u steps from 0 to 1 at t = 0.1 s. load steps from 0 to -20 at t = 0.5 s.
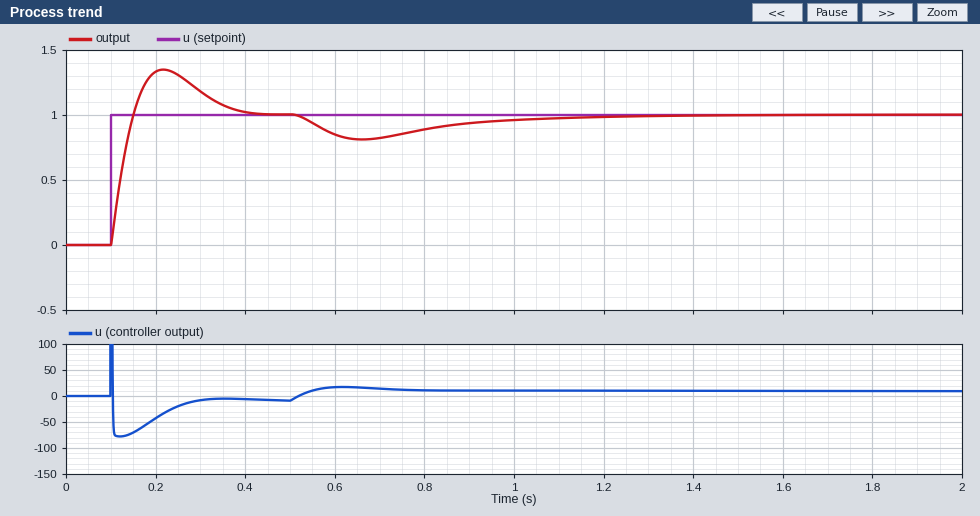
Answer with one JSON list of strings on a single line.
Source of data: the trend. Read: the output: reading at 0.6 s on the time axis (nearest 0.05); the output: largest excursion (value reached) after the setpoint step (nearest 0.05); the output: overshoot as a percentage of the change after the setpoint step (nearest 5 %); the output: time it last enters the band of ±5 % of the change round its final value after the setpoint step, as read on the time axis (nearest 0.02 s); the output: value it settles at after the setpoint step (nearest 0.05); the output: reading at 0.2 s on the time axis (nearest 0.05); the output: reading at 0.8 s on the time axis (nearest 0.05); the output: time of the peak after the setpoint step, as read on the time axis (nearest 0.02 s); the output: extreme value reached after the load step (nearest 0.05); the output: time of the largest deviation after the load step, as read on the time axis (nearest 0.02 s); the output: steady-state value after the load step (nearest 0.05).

["0.85", "1.35", "35 %", "0.36 s", "1.00", "1.35", "0.90", "0.22 s", "0.80", "0.66 s", "1.00"]
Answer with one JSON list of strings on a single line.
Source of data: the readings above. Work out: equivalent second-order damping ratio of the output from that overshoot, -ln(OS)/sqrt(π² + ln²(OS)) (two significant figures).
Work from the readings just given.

["0.32"]
